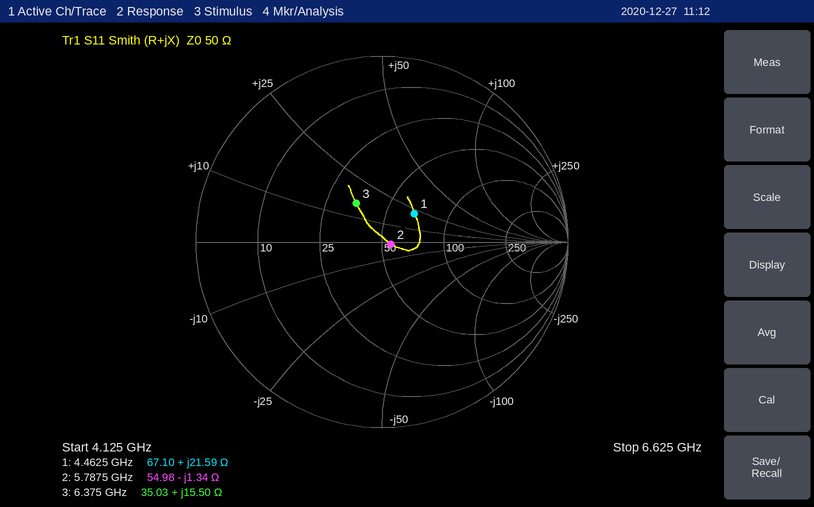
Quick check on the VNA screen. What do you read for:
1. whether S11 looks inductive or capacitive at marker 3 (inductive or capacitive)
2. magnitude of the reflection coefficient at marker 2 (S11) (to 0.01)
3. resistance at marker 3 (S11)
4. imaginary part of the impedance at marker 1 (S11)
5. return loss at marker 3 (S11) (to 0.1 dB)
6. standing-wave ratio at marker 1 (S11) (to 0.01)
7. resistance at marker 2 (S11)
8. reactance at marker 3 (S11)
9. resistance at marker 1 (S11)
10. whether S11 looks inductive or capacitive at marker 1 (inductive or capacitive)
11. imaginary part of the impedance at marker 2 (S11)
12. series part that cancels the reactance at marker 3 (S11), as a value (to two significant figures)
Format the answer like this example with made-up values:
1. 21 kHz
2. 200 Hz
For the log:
1. inductive
2. 0.05
3. 35.03 Ω
4. +21.59 Ω
5. 12.1 dB
6. 1.60
7. 54.98 Ω
8. +15.50 Ω
9. 67.10 Ω
10. inductive
11. -1.34 Ω
12. 1.6 pF
